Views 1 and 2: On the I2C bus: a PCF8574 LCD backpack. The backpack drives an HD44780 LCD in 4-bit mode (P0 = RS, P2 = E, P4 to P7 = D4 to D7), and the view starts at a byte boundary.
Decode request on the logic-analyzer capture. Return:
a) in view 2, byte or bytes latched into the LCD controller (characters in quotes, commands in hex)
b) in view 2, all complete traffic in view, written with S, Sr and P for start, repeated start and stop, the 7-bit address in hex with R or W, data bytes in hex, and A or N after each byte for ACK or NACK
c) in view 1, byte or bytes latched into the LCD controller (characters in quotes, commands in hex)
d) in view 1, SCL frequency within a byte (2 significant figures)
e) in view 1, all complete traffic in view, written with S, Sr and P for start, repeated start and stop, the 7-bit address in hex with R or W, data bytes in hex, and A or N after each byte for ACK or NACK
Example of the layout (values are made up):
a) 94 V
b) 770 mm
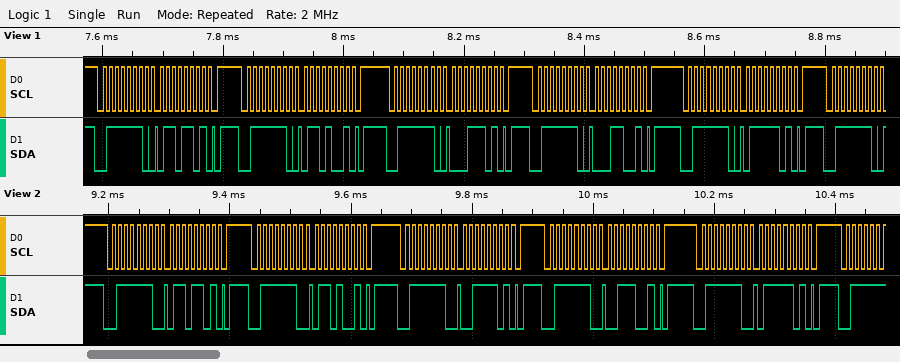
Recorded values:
a) 'c'
b) S 3FW A 6D A P S 3FW A 69 A P S 3FW A 3D A P S 3FW A 39 A P S 3FW A 7D A P
c) 'a'
d) 100 kHz
e) S 3FW A 6D A P S 3FW A 69 A P S 3FW A 1D A P S 3FW A 19 A P S 3FW A 7D A P S 3FW A
